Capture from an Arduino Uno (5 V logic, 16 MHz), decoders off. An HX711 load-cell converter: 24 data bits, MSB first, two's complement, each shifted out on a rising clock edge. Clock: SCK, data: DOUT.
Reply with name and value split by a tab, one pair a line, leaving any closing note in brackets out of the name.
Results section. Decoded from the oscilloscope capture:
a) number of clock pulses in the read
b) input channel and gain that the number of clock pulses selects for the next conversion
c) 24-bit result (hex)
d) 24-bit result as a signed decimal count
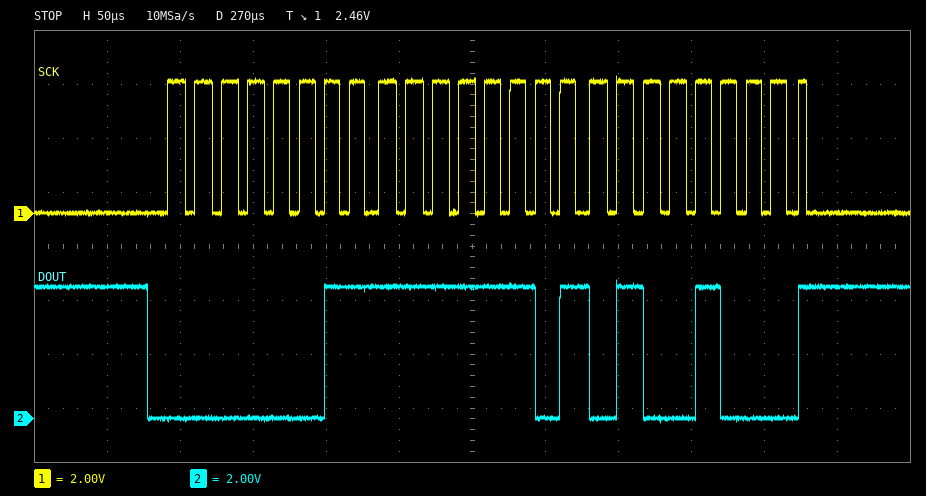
number of clock pulses in the read	25
input channel and gain that the number of clock pulses selects for the next conversion	channel A, gain 128
24-bit result	0x03FD48
24-bit result as a signed decimal count	261448
